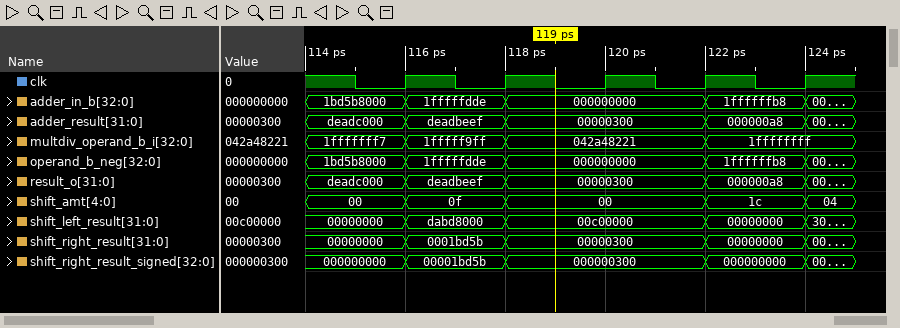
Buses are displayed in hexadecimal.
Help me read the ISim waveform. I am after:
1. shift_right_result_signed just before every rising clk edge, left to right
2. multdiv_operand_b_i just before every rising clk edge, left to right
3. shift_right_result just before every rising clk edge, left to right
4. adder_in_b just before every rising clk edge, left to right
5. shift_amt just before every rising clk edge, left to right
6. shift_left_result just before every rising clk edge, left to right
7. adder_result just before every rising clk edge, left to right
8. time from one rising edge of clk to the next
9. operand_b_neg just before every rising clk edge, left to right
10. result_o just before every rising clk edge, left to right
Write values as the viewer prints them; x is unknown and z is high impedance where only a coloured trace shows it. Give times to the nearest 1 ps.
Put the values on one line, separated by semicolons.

000000000, 00001bd5b, 000000300, 000000300, 000000000; 1fffffff7, 1fffff9ff, 042a48221, 042a48221, 1ffffffff; 00000000, 0001bd5b, 00000300, 00000300, 00000000; 1bd5b8000, 1fffffdde, 000000000, 000000000, 1ffffffb8; 00, 0f, 00, 00, 1c; 00000000, dabd8000, 00c00000, 00c00000, 00000000; deadc000, deadbeef, 00000300, 00000300, 000000a8; 2 ps; 1bd5b8000, 1fffffdde, 000000000, 000000000, 1ffffffb8; deadc000, deadbeef, 00000300, 00000300, 000000a8
